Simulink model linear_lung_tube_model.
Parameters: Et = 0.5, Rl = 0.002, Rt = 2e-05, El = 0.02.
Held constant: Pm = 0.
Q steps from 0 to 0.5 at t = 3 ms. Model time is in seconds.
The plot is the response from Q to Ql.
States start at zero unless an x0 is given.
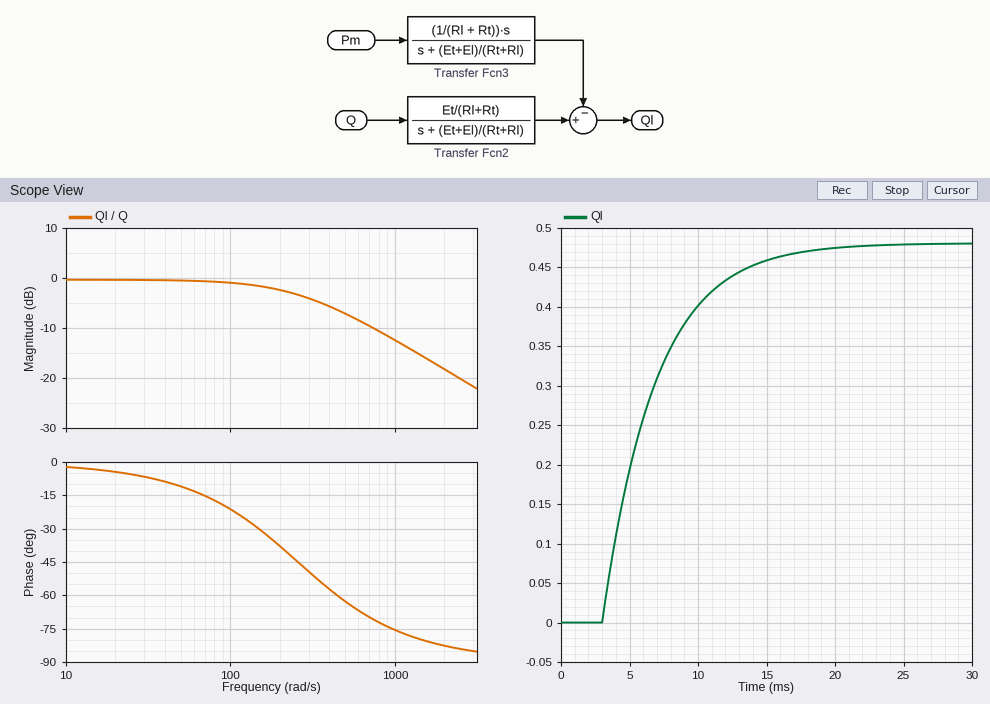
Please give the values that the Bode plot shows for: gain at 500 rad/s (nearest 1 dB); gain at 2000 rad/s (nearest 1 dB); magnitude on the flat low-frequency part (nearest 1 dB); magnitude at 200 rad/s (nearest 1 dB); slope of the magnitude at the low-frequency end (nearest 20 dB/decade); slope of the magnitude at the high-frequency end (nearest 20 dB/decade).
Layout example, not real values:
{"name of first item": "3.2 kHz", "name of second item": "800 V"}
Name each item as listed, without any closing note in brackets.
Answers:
{"gain at 500 rad/s": "-7 dB", "gain at 2000 rad/s": "-18 dB", "magnitude on the flat low-frequency part": "0 dB", "magnitude at 200 rad/s": "-2 dB", "slope of the magnitude at the low-frequency end": "0 dB/decade", "slope of the magnitude at the high-frequency end": "-20 dB/decade"}
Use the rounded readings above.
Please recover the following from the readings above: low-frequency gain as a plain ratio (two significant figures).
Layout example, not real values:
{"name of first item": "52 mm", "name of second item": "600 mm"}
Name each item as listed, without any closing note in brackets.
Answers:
{"low-frequency gain as a plain ratio": "1.0"}
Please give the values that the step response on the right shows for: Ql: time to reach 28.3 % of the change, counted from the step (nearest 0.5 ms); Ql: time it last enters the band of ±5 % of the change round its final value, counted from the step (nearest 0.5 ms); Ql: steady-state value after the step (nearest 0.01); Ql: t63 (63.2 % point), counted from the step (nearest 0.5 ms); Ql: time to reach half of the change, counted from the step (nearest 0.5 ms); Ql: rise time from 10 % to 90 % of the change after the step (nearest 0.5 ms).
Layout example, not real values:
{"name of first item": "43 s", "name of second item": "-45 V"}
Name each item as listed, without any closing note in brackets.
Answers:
{"Ql: time to reach 28.3 % of the change, counted from the step": "1.5 ms", "Ql: time it last enters the band of ±5 % of the change round its final value, counted from the step": "11.5 ms", "Ql: steady-state value after the step": "0.48", "Ql: t63 (63.2 % point), counted from the step": "4.0 ms", "Ql: time to reach half of the change, counted from the step": "2.5 ms", "Ql: rise time from 10 % to 90 % of the change after the step": "8.5 ms"}
